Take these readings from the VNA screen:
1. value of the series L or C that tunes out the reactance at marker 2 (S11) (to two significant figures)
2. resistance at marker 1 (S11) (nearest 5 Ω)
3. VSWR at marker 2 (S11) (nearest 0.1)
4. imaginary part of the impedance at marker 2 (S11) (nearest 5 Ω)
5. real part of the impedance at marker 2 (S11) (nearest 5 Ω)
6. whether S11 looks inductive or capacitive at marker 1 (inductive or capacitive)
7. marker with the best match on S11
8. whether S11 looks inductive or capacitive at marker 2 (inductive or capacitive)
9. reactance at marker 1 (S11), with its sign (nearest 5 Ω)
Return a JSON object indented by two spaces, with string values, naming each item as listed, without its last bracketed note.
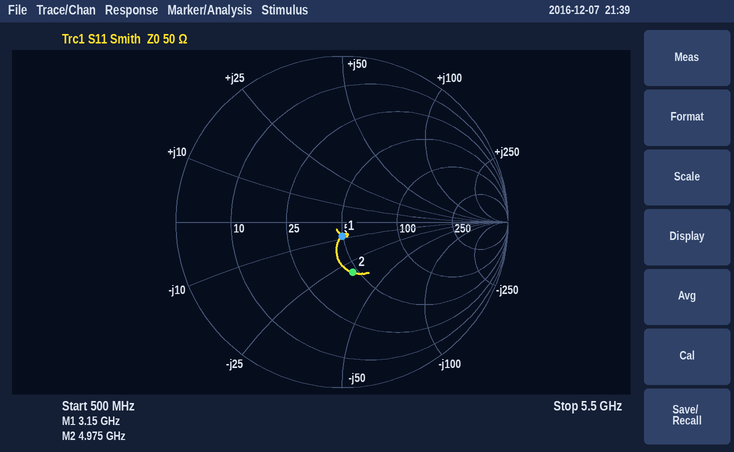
{
  "value of the series L or C that tunes out the reactance at marker 2 (S11)": "1.0 nH",
  "resistance at marker 1 (S11)": "50 Ω",
  "VSWR at marker 2 (S11)": "1.9",
  "imaginary part of the impedance at marker 2 (S11)": "-30 Ω",
  "real part of the impedance at marker 2 (S11)": "45 Ω",
  "whether S11 looks inductive or capacitive at marker 1": "capacitive",
  "marker with the best match on S11": "marker 1",
  "whether S11 looks inductive or capacitive at marker 2": "capacitive",
  "reactance at marker 1 (S11), with its sign": "-10 Ω"
}
